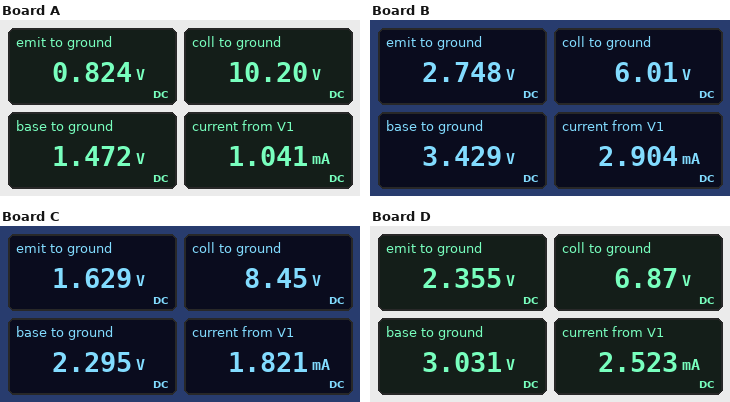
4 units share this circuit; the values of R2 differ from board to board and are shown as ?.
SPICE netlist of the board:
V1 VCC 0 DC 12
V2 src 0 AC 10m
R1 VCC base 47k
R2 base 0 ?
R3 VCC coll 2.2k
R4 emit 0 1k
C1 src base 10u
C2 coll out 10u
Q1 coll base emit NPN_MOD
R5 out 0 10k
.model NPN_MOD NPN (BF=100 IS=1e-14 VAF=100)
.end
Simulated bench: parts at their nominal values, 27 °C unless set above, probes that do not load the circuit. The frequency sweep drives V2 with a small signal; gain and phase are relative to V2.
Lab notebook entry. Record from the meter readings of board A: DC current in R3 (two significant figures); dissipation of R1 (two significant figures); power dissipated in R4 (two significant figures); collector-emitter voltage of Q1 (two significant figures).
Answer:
820 µA
2.4 mW
680 µW
9.4 V
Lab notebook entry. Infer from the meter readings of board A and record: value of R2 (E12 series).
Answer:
6.8 kΩ
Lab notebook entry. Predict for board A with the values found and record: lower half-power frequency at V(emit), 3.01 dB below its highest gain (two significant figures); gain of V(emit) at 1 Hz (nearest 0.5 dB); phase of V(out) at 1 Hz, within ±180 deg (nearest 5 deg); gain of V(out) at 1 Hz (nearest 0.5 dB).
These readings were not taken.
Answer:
2.8 Hz
-10.0 dB
-55 deg
-9.0 dB
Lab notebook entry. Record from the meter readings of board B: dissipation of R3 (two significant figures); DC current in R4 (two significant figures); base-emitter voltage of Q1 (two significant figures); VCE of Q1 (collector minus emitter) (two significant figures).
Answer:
16 mW
2.7 mA
680 mV
3.3 V
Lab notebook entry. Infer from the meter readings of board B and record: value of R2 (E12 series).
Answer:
22 kΩ
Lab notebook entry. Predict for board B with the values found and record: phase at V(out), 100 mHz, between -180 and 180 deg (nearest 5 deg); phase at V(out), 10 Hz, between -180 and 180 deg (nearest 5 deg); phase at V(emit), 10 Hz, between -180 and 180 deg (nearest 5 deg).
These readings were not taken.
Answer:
-10 deg
-165 deg
5 deg
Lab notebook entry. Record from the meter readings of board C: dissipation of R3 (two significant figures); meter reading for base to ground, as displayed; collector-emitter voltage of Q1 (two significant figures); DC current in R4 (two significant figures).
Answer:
5.7 mW
2.295 V
6.8 V
1.6 mA
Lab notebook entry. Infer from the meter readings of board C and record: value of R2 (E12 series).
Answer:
12 kΩ
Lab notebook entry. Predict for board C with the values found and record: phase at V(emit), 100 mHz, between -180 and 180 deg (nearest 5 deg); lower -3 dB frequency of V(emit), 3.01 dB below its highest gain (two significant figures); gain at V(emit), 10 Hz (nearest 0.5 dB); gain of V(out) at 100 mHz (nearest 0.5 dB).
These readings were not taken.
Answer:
85 deg
1.8 Hz
-0.5 dB
-42.5 dB
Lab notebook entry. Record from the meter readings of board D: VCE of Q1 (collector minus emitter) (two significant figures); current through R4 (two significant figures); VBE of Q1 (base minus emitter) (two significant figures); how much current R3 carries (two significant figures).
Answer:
4.5 V
2.4 mA
680 mV
2.3 mA
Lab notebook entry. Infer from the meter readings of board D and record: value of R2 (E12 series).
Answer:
18 kΩ
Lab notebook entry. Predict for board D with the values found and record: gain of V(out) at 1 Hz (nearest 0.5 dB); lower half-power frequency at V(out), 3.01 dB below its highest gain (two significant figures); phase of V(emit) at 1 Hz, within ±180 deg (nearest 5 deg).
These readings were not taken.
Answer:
-4.0 dB
2.1 Hz
55 deg
